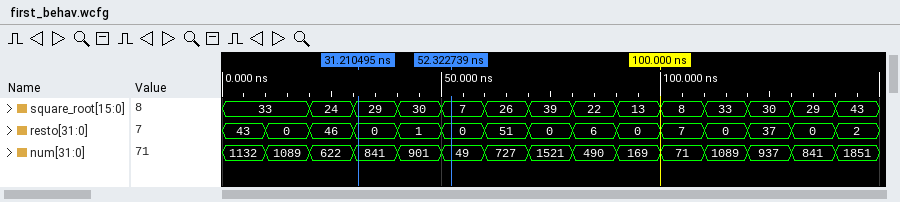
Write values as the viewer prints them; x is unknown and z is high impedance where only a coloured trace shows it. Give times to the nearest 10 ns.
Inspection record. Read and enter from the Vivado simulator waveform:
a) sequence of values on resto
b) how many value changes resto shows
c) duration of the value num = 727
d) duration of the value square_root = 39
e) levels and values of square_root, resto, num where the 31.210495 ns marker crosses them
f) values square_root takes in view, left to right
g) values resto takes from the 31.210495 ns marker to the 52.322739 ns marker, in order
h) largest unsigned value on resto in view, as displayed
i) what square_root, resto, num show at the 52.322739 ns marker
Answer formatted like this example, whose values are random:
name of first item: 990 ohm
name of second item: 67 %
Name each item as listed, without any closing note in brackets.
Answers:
sequence of values on resto: 43, 0, 46, 0, 1, 0, 51, 0, 6, 0, 7, 0, 37, 0, 2
how many value changes resto shows: 14
duration of the value num = 727: 10 ns
duration of the value square_root = 39: 10 ns
levels and values of square_root, resto, num where the 31.210495 ns marker crosses them: square_root=29, resto=0, num=841
values square_root takes in view, left to right: 33, 24, 29, 30, 7, 26, 39, 22, 13, 8, 33, 30, 29, 43
values resto takes from the 31.210495 ns marker to the 52.322739 ns marker, in order: 0, 1, 0
largest unsigned value on resto in view, as displayed: 51
what square_root, resto, num show at the 52.322739 ns marker: square_root=7, resto=0, num=49
